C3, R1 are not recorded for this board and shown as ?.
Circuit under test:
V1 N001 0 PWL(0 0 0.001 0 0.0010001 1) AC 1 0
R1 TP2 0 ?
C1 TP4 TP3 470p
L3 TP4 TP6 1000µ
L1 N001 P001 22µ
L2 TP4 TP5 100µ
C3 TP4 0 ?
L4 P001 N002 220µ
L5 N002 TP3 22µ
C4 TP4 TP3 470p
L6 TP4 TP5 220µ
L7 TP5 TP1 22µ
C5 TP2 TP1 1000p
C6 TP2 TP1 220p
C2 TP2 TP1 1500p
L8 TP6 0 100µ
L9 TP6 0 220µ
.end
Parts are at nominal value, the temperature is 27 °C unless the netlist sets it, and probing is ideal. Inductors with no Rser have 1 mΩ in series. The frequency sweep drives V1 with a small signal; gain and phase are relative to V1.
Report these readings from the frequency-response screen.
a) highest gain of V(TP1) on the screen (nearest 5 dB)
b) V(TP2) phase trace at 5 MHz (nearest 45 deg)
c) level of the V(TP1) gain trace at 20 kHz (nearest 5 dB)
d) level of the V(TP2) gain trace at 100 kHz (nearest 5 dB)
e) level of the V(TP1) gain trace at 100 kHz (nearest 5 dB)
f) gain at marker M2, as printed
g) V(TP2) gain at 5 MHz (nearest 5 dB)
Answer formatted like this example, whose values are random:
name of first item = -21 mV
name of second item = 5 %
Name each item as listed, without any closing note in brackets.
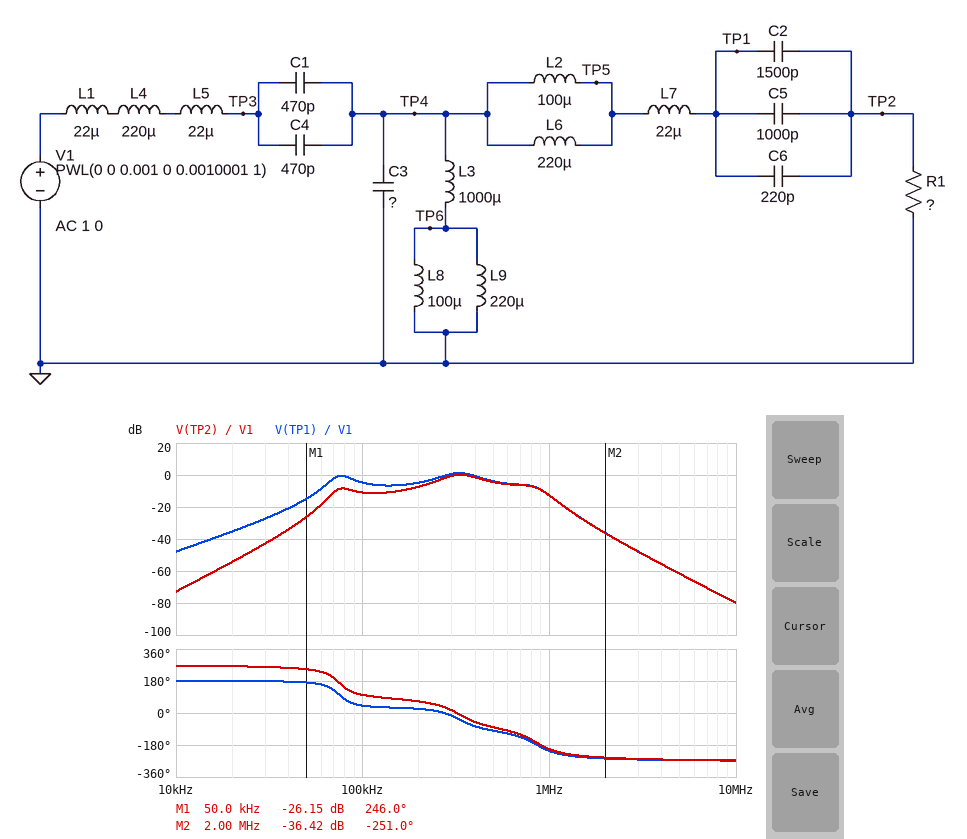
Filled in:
highest gain of V(TP1) on the screen = 0 dB
V(TP2) phase trace at 5 MHz = -270 deg
level of the V(TP1) gain trace at 20 kHz = -35 dB
level of the V(TP2) gain trace at 100 kHz = -10 dB
level of the V(TP1) gain trace at 100 kHz = -5 dB
gain at marker M2, as printed = -36.42 dB
V(TP2) gain at 5 MHz = -60 dB
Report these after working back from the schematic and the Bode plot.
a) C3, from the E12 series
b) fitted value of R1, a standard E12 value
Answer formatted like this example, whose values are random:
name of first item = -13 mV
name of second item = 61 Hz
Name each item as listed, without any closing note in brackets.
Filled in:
C3, from the E12 series = 560 pF
fitted value of R1, a standard E12 value = 330 Ω
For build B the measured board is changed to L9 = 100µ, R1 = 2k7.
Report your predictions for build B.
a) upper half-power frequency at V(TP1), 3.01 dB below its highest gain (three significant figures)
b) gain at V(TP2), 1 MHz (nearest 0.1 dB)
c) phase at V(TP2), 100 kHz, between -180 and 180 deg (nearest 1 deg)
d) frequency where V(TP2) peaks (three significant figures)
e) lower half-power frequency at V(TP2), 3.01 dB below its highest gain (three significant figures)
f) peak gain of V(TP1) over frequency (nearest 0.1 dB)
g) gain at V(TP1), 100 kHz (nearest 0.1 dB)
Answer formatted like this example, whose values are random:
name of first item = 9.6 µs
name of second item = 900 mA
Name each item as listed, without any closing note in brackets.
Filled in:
upper half-power frequency at V(TP1), 3.01 dB below its highest gain = 583 kHz
gain at V(TP2), 1 MHz = -12.1 dB
phase at V(TP2), 100 kHz, between -180 and 180 deg = 152 deg
frequency where V(TP2) peaks = 547 kHz
lower half-power frequency at V(TP2), 3.01 dB below its highest gain = 508 kHz
peak gain of V(TP1) over frequency = 13.0 dB
gain at V(TP1), 100 kHz = 1.3 dB
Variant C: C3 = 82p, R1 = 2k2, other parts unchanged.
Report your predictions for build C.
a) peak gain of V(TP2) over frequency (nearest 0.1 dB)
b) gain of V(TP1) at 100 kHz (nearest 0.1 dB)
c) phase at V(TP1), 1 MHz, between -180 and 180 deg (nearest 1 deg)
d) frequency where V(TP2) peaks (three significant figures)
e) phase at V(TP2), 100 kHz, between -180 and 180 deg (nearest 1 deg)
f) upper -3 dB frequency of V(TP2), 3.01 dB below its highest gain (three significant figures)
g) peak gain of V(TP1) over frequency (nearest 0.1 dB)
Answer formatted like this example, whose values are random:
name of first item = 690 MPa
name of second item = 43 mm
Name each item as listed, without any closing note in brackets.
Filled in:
peak gain of V(TP2) over frequency = 6.9 dB
gain of V(TP1) at 100 kHz = -1.7 dB
phase at V(TP1), 1 MHz, between -180 and 180 deg = -61 deg
frequency where V(TP2) peaks = 141 kHz
phase at V(TP2), 100 kHz, between -180 and 180 deg = 161 deg
upper -3 dB frequency of V(TP2), 3.01 dB below its highest gain = 181 kHz
peak gain of V(TP1) over frequency = 7.1 dB
